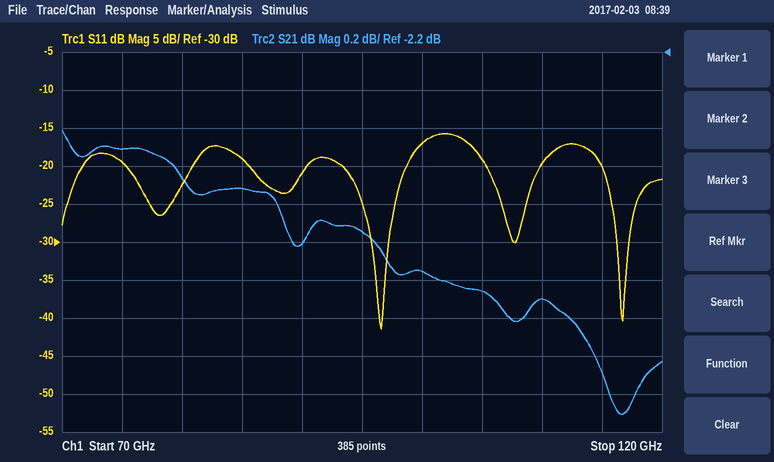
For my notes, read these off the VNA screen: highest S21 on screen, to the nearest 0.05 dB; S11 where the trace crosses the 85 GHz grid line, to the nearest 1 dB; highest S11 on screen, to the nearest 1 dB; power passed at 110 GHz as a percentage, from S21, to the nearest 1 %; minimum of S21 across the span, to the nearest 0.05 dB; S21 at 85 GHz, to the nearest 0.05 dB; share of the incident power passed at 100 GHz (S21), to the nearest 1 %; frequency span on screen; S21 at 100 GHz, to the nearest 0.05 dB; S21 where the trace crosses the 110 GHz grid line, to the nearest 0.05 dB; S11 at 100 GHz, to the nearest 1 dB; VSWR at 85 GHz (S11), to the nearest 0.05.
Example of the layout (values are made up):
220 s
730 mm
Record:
-2.60 dB
-19 dB
-16 dB
45 %
-4.10 dB
-2.90 dB
46 %
50 GHz
-3.35 dB
-3.50 dB
-17 dB
1.25
